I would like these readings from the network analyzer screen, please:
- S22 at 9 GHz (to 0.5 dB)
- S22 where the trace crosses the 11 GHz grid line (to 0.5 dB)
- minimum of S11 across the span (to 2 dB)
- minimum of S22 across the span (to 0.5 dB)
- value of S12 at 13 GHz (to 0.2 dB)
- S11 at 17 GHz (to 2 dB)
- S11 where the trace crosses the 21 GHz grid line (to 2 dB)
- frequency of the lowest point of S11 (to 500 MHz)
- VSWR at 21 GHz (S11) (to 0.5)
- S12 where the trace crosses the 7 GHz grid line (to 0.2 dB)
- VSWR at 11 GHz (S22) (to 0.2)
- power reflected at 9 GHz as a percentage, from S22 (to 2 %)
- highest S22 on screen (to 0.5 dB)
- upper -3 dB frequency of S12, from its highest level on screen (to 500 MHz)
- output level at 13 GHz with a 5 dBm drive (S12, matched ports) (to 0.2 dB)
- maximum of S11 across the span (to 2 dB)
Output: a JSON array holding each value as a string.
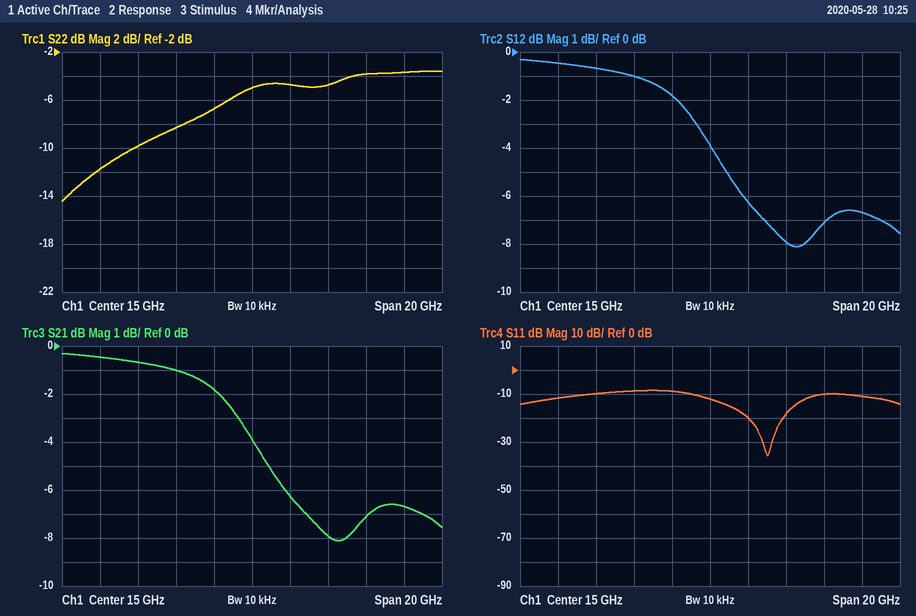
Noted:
["-10.0 dB", "-8.5 dB", "-36 dB", "-14.5 dB", "-1.8 dB", "-20 dB", "-10 dB", "18.0 GHz", "2.0", "-0.4 dB", "2.2", "10 %", "-3.5 dB", "14.5 GHz", "3.2 dBm", "-8 dB"]
